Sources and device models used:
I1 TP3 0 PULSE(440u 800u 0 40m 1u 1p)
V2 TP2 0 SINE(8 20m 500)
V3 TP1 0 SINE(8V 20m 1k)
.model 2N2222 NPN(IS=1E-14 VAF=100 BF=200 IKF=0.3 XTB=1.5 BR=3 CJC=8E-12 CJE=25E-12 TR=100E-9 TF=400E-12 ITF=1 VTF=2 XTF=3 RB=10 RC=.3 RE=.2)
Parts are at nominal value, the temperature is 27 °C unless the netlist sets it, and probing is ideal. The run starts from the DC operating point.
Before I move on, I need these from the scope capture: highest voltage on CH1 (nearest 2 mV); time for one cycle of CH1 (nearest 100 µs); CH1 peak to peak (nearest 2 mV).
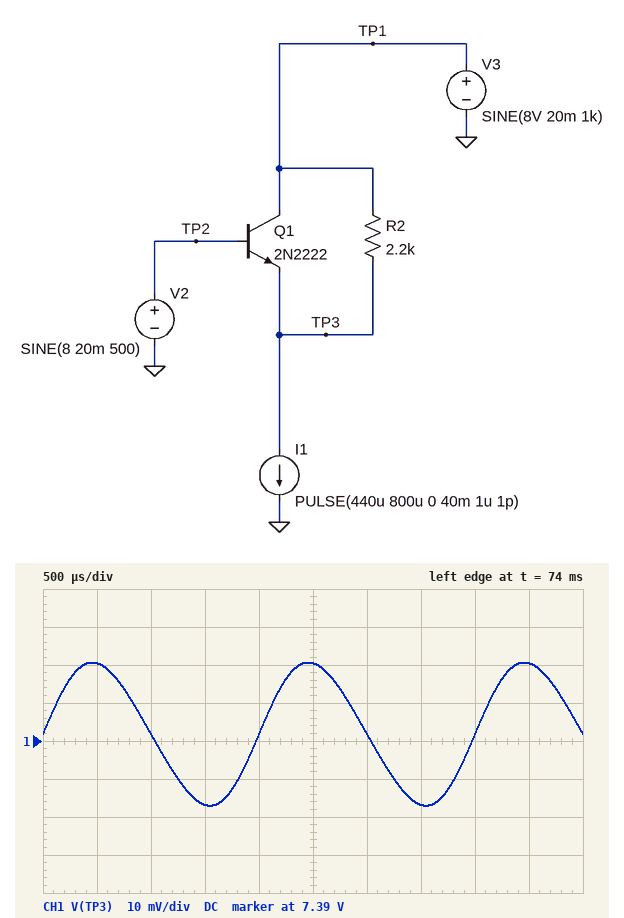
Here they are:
7.410 V
2.0 ms
38 mV
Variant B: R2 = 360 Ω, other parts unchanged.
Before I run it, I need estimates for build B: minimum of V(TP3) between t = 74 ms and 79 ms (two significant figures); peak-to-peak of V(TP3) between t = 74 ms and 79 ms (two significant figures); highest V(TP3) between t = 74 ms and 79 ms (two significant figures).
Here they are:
7.8 V
40 mV
7.9 V
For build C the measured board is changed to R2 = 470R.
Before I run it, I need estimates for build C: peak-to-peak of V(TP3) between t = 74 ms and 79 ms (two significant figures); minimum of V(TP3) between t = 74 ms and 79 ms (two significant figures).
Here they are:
40 mV
7.8 V
